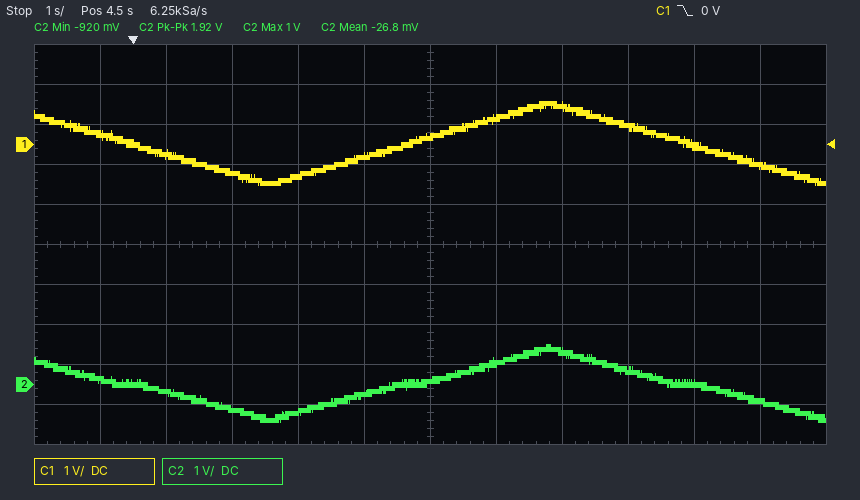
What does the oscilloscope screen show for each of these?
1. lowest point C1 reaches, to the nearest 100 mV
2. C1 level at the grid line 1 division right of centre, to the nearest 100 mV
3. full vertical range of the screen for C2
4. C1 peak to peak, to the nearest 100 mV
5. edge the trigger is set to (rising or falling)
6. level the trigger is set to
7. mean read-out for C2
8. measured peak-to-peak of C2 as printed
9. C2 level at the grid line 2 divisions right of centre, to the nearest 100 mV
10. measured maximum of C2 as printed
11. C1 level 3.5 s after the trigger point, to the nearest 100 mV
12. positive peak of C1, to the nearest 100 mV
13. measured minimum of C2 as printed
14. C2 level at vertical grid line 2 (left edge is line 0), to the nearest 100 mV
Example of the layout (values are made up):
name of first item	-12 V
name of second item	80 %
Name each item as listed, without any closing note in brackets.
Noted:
lowest point C1 reaches, to the nearest 100 mV	-1.0 V
C1 level at the grid line 1 division right of centre, to the nearest 100 mV	700 mV
full vertical range of the screen for C2	10 V
C1 peak to peak, to the nearest 100 mV	2.1 V
edge the trigger is set to	falling
level the trigger is set to	0 V
mean read-out for C2	-26.8 mV
measured peak-to-peak of C2 as printed	1.92 V
C2 level at the grid line 2 divisions right of centre, to the nearest 100 mV	800 mV
measured maximum of C2 as printed	1 V
C1 level 3.5 s after the trigger point, to the nearest 100 mV	-300 mV
positive peak of C1, to the nearest 100 mV	1.1 V
measured minimum of C2 as printed	-920 mV
C2 level at vertical grid line 2 (left edge is line 0), to the nearest 100 mV	-200 mV
